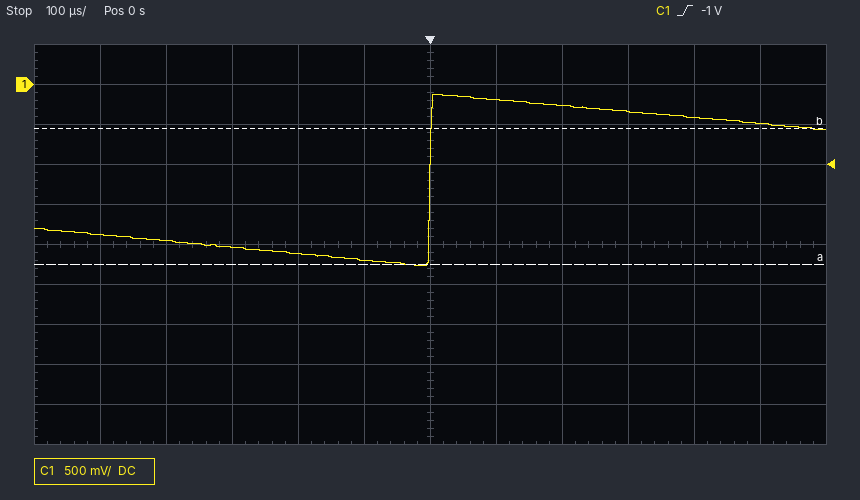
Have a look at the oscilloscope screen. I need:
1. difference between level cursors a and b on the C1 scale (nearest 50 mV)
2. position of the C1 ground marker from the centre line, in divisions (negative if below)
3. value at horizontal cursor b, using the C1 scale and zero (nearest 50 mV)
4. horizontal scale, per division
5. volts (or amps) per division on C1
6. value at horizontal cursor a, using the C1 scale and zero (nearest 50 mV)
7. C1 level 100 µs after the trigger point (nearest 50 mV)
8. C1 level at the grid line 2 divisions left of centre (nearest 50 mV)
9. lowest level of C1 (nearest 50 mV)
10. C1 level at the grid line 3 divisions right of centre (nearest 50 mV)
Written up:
1.70 V
+4.0 div
-550 mV
100 µs
500 mV
-2.25 V
-200 mV
-2.10 V
-2.25 V
-350 mV
